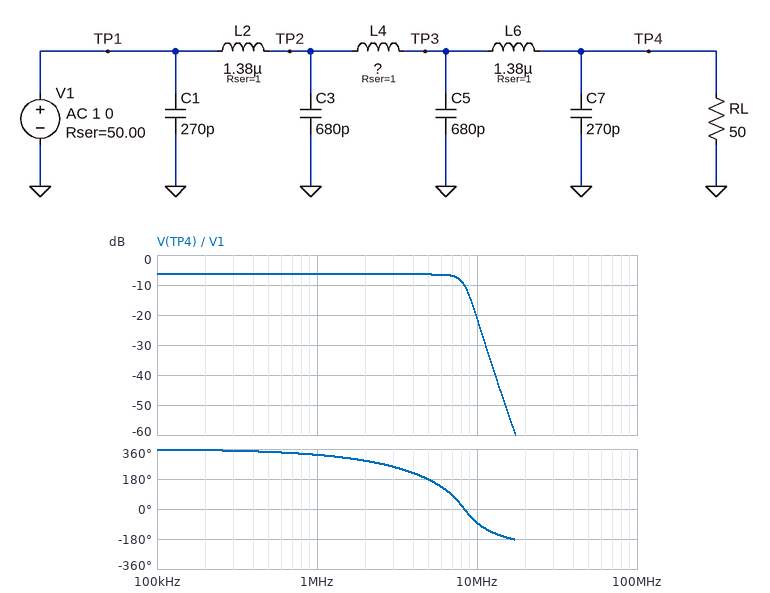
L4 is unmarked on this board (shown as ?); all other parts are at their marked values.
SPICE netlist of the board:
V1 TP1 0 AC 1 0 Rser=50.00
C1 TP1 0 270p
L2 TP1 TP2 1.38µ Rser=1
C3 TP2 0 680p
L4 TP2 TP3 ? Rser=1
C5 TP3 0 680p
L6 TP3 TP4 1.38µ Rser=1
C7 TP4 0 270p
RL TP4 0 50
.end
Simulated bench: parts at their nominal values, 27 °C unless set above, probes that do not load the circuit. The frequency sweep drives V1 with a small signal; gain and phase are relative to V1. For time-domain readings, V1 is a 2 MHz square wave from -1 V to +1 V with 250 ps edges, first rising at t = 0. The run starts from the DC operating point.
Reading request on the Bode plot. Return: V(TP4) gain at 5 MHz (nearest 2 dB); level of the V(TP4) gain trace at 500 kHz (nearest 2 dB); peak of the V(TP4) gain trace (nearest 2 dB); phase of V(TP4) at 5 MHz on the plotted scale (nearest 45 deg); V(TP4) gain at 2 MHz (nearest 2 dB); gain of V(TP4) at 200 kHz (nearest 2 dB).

-6 dB
-6 dB
-6 dB
180 deg
-6 dB
-6 dB
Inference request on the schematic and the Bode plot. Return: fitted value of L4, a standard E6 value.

2.2 µH
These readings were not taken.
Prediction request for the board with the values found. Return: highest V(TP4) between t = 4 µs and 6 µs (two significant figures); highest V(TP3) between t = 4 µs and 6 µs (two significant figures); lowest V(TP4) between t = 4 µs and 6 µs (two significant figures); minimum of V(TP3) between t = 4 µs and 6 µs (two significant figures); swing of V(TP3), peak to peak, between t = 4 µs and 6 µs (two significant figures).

630 mV
660 mV
-630 mV
-660 mV
1.3 V
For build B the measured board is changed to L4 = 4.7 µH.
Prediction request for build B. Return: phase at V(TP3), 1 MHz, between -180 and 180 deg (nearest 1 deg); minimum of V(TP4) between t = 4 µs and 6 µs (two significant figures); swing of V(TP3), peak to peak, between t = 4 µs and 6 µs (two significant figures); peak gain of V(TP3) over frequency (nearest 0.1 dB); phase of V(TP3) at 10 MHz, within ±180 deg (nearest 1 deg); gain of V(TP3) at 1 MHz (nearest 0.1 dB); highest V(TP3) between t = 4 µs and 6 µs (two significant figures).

-34 deg
-510 mV
1.0 V
-6.1 dB
13 deg
-6.2 dB
510 mV
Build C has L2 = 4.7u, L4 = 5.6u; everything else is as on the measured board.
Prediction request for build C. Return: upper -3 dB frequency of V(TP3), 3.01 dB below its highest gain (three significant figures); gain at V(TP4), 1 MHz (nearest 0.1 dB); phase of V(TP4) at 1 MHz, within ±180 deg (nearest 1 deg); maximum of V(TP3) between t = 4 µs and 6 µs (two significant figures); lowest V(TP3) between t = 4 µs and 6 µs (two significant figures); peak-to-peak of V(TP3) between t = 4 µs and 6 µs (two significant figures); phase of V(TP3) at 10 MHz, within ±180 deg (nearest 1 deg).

4.53 MHz
-6.9 dB
-57 deg
510 mV
-510 mV
1.0 V
-20 deg
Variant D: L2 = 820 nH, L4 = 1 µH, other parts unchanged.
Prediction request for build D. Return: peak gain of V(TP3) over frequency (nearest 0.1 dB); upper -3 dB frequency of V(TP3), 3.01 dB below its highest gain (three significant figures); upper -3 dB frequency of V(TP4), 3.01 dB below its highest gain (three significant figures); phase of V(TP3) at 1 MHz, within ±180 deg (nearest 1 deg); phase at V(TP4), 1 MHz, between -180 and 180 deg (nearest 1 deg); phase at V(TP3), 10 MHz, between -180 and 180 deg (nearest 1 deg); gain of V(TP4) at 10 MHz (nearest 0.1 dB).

-2.6 dB
11.5 MHz
10.7 MHz
-19 deg
-29 deg
134 deg
-7.8 dB
